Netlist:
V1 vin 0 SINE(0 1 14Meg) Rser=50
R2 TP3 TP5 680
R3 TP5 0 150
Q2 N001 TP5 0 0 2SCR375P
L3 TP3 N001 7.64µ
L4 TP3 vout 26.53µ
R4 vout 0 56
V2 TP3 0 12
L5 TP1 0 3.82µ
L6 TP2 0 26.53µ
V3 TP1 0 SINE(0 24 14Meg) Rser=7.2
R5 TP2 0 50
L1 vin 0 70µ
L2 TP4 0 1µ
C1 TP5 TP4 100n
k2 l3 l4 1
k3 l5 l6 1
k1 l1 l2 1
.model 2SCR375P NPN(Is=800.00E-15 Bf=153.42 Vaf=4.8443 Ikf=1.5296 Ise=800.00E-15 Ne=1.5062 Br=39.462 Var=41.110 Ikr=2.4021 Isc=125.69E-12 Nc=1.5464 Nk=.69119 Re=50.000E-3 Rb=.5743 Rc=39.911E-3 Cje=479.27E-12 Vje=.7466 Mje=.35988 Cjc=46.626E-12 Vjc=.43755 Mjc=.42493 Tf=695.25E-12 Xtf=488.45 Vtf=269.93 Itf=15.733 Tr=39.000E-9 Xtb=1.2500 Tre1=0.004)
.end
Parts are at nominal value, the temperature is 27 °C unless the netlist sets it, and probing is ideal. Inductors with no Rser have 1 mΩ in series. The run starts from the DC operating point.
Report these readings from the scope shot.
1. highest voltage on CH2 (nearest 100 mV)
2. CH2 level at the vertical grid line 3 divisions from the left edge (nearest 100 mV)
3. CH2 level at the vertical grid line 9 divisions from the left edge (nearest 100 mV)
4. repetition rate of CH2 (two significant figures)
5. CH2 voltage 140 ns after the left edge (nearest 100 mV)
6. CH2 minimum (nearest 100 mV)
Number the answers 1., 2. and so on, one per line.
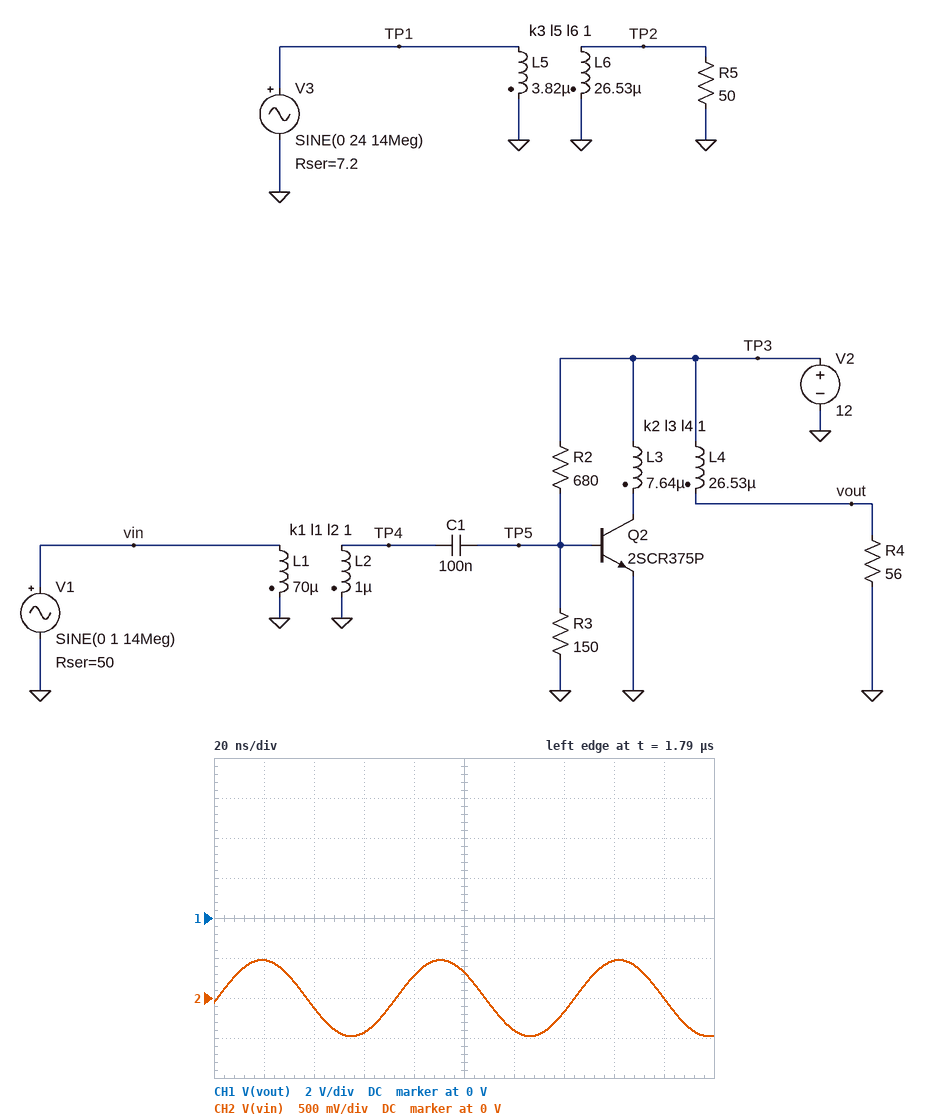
1. 500 mV
2. -400 mV
3. 0 V
4. 14 MHz
5. -200 mV
6. -500 mV
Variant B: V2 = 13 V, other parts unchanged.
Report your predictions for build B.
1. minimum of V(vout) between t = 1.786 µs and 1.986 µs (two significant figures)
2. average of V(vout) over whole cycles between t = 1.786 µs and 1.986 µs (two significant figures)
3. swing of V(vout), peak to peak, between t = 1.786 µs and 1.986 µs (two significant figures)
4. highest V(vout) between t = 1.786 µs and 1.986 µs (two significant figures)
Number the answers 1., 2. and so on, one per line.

1. 12 V
2. 13 V
3. 1.3 V
4. 14 V
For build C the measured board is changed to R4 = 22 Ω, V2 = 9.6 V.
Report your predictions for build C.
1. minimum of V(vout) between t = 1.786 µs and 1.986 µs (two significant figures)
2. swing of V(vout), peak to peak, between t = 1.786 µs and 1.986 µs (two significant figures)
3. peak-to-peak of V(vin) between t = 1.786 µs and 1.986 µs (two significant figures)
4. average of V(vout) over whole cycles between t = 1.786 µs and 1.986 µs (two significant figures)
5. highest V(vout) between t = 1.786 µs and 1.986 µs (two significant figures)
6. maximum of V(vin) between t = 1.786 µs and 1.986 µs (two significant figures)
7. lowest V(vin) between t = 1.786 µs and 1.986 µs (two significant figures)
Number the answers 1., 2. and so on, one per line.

1. 8.6 V
2. 2.3 V
3. 970 mV
4. 9.6 V
5. 11 V
6. 490 mV
7. -490 mV
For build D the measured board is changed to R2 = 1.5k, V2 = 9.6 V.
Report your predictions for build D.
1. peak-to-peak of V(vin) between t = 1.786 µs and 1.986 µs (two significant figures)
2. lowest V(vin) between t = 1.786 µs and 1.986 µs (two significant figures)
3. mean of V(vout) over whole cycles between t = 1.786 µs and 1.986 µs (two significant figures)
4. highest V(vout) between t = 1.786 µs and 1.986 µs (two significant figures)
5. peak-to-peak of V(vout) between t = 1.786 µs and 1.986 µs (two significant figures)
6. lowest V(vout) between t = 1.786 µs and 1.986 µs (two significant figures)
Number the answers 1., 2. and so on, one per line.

1. 1.7 V
2. -950 mV
3. 10 V
4. 22 V
5. 23 V
6. -380 mV
